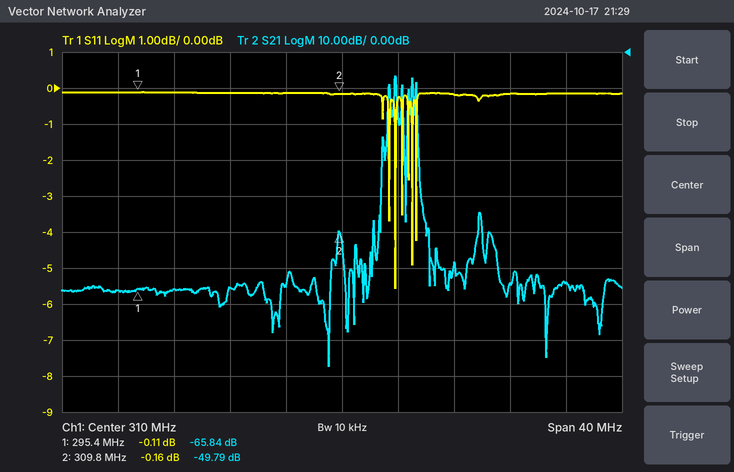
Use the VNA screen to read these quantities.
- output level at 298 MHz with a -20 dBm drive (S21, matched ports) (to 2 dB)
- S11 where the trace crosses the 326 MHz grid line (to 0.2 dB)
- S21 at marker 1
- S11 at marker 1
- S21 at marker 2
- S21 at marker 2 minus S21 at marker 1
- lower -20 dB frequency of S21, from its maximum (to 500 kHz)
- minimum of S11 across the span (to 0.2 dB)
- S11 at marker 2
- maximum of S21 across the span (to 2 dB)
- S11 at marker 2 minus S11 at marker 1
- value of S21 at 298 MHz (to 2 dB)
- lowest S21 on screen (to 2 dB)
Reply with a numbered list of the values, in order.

1. -86 dBm
2. -0.2 dB
3. -65.84 dB
4. -0.11 dB
5. -49.79 dB
6. 16.05 dB
7. 313.0 MHz
8. -5.6 dB
9. -0.16 dB
10. -6 dB
11. -0.05 dB
12. -66 dB
13. -88 dB
